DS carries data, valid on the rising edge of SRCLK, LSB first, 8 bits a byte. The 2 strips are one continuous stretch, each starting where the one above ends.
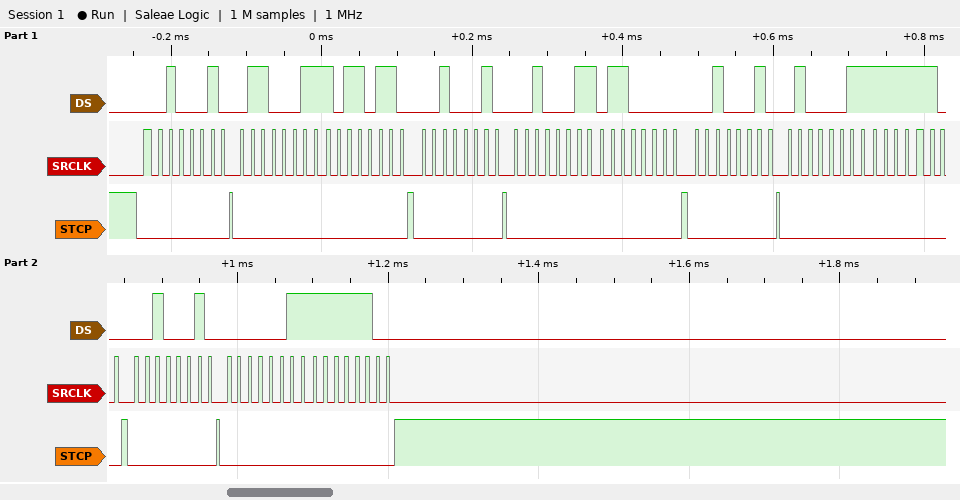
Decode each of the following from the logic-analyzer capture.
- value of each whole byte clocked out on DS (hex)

44 C6 6D 44 C4 06 44 C2 3F 44 C0 3F
